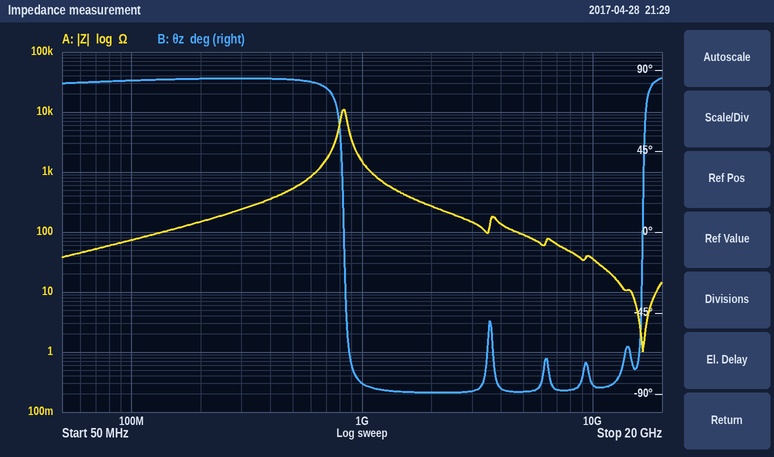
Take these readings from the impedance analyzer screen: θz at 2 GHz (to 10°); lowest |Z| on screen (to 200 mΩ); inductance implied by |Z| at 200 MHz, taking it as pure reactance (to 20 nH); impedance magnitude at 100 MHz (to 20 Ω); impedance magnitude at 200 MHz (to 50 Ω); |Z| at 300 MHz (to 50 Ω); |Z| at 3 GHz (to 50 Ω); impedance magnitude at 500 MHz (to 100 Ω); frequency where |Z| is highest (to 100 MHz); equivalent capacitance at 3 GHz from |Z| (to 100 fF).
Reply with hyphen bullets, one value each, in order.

- -90°
- 1.0 Ω
- 120 nH
- 80 Ω
- 150 Ω
- 250 Ω
- 150 Ω
- 500 Ω
- 800 MHz
- 400 fF
